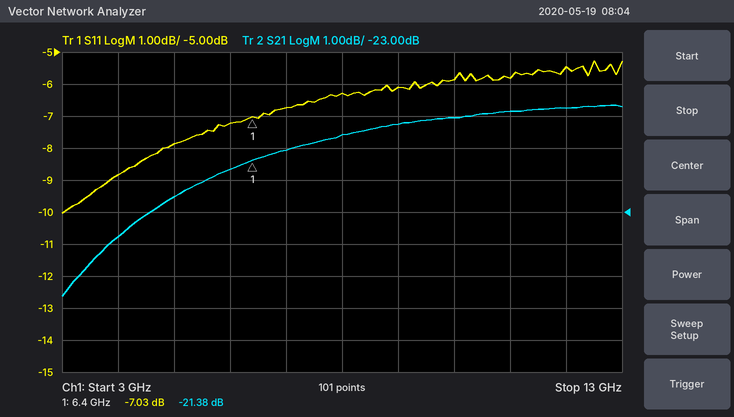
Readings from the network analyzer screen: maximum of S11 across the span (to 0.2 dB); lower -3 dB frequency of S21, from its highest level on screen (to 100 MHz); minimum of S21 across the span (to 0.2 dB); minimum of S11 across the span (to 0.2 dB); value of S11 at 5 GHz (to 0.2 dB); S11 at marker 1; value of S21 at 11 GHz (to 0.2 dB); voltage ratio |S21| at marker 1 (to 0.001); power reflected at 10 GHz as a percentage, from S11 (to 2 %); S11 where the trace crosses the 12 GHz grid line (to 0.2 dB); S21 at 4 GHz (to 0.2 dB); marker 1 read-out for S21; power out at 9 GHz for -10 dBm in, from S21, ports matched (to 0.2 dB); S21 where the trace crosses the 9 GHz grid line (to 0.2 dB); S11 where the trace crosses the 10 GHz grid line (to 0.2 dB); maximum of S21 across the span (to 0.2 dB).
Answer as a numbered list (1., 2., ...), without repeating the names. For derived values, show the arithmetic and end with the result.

1. -5.2 dB
2. 4.9 GHz
3. -25.6 dB
4. -10.0 dB
5. -7.8 dB
6. -7.03 dB
7. -19.8 dB
8. 10^(-21.38/20) ≈ 0.085
9. 10^(-5.8/10) ≈ 26 %
10. -5.4 dB
11. -23.8 dB
12. -21.38 dB
13. -10 dBm + (-20.2 dB) = -30.2 dBm
14. -20.2 dB
15. -5.8 dB
16. -19.6 dB
